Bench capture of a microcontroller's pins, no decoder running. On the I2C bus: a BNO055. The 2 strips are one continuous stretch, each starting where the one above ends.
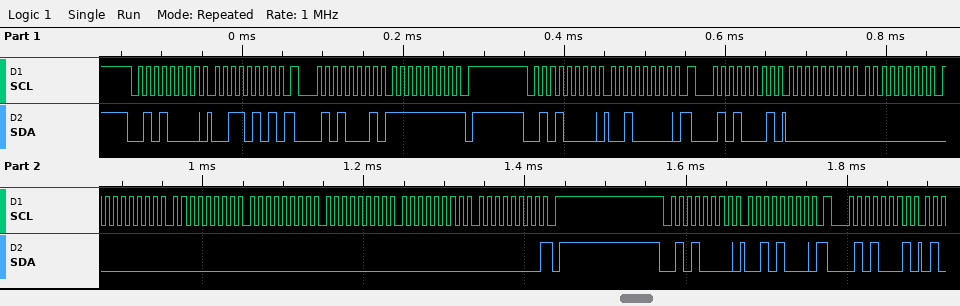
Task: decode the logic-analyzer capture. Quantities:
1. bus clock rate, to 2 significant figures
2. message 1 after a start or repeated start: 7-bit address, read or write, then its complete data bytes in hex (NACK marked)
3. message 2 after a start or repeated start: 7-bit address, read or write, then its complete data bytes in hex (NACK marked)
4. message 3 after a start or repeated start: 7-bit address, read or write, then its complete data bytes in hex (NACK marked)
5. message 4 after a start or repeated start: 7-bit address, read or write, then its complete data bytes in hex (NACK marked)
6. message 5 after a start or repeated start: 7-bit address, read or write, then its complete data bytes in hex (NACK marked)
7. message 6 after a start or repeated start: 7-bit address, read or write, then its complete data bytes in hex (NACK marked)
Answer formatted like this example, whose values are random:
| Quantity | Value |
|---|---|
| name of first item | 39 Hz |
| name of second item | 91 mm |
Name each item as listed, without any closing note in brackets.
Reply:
| Quantity | Value |
|---|---|
| bus clock rate, to 2 significant figures | 100 kHz |
| message 1 after a start or repeated start: 7-bit address, read or write, then its complete data bytes in hex | 0x28 write: 35 |
| message 2 after a start or repeated start: 7-bit address, read or write, then its complete data bytes in hex | 0x28 read: FF NACK |
| message 3 after a start or repeated start: 7-bit address, read or write, then its complete data bytes in hex | 0x28 write: 20 |
| message 4 after a start or repeated start: 7-bit address, read or write, then its complete data bytes in hex | 0x28 read: 00 00 00 00 00 00 00 00 NACK |
| message 5 after a start or repeated start: 7-bit address, read or write, then its complete data bytes in hex | 0x28 write: 28 |
| message 6 after a start or repeated start: 7-bit address, read or write, then its complete data bytes in hex | 0x28 read |
